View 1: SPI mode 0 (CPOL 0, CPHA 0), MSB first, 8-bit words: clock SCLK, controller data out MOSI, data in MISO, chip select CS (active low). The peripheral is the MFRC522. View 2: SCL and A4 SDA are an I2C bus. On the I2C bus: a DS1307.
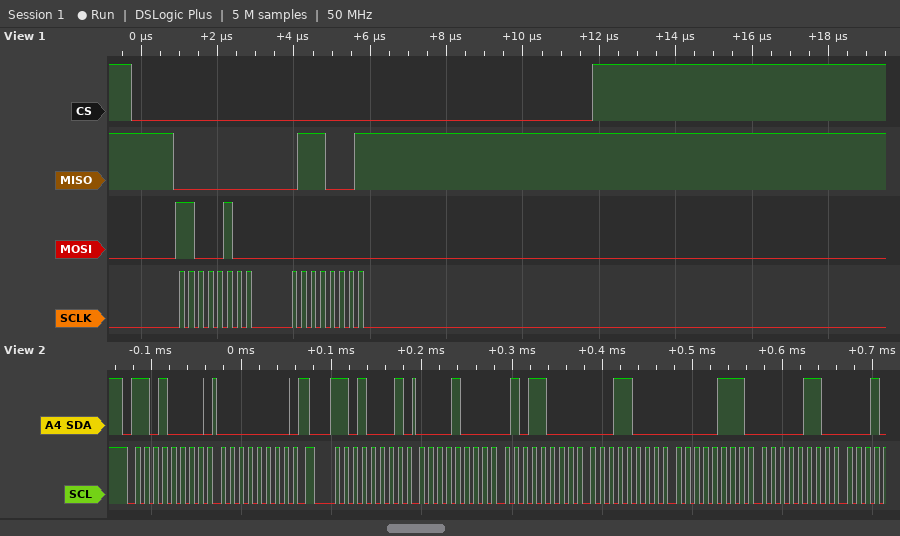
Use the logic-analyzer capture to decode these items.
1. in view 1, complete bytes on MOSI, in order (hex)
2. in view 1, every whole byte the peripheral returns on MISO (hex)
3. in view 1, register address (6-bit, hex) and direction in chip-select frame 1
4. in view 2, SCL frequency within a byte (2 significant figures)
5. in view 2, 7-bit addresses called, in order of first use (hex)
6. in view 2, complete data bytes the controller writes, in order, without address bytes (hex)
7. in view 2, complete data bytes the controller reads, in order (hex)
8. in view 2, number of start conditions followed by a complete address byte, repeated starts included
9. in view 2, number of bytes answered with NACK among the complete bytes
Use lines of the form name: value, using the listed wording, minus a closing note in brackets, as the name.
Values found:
in view 1, complete bytes on MOSI, in order: 0xC4 0x00
in view 1, every whole byte the peripheral returns on MISO: 0x00 0x71
in view 1, register address (6-bit, hex) and direction in chip-select frame 1: 0x22 read
in view 2, SCL frequency within a byte: 100 kHz
in view 2, 7-bit addresses called, in order of first use: 0x68
in view 2, complete data bytes the controller writes, in order, without address bytes: 00
in view 2, complete data bytes the controller reads, in order: 08 58 18 07 06
in view 2, number of start conditions followed by a complete address byte, repeated starts included: 2
in view 2, number of bytes answered with NACK among the complete bytes: 0
